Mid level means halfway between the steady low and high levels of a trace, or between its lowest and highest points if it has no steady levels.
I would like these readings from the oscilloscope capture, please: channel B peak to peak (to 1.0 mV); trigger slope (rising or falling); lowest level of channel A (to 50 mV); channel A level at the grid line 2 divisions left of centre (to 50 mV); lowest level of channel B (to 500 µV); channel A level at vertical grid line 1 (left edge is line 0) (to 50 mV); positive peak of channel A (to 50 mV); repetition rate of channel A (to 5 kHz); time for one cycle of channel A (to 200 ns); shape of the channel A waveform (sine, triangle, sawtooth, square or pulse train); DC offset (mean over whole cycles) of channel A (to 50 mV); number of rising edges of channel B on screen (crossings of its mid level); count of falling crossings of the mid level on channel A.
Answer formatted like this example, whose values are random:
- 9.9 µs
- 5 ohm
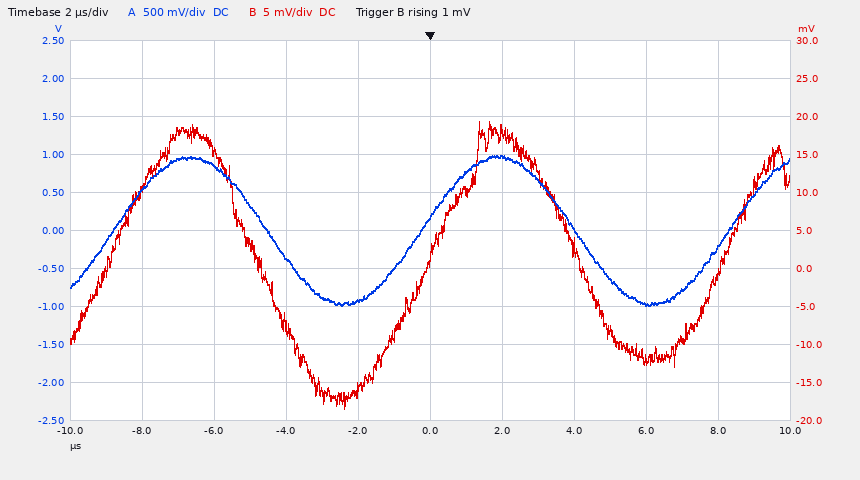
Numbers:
- 38.0 mV
- rising
- -1.00 V
- -350 mV
- -18.5 mV
- 550 mV
- 1.00 V
- 115 kHz
- 8.6 µs
- sine
- 0 mV
- 3
- 2
